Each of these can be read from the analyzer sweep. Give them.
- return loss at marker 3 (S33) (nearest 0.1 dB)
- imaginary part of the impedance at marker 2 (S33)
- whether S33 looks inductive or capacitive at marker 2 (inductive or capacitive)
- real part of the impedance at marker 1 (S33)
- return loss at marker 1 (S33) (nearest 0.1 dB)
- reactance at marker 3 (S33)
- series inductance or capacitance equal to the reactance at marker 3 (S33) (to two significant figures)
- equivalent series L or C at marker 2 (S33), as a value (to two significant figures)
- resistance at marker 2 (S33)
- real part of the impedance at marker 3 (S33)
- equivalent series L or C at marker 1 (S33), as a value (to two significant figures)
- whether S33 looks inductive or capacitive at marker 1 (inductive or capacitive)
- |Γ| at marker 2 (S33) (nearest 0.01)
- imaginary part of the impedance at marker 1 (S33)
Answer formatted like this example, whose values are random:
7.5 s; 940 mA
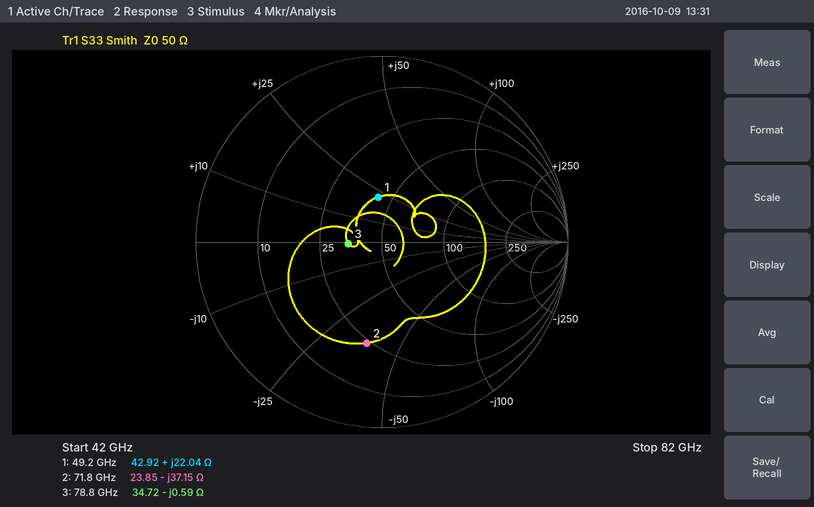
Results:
14.9 dB; -37.15 Ω; capacitive; 42.92 Ω; 12.3 dB; -0.59 Ω; 3.4 pF; 60 fF; 23.85 Ω; 34.72 Ω; 71 pH; inductive; 0.55; +22.04 Ω
